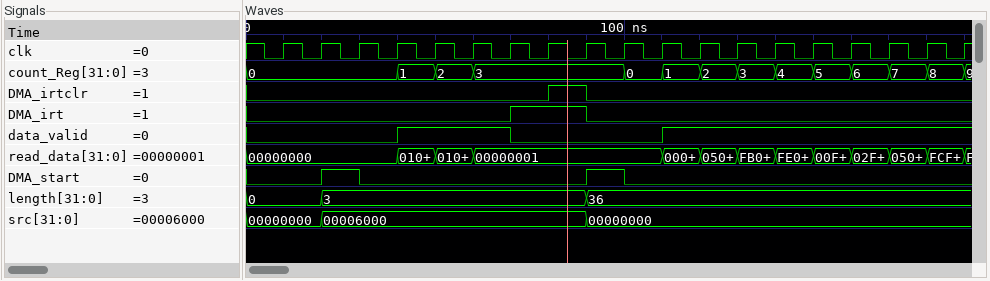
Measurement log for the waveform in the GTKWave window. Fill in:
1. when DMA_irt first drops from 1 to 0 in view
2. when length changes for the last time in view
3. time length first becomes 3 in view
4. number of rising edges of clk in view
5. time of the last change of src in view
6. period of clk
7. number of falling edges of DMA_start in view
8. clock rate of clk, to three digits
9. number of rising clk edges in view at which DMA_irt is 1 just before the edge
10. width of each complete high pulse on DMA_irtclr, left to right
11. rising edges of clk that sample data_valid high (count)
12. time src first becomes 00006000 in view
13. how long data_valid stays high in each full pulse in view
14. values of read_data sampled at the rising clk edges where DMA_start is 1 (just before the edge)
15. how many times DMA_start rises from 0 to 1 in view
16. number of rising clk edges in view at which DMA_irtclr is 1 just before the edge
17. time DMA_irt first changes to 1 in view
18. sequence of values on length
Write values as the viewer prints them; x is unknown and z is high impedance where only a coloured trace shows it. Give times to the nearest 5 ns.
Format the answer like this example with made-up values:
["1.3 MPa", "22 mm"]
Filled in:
["90 ns", "90 ns", "20 ns", "19", "90 ns", "10 ns", "2", "100 MHz", "2", "10 ns", "11", "20 ns", "30 ns", "00000000, 00000001", "2", "1", "70 ns", "0, 3, 36"]
